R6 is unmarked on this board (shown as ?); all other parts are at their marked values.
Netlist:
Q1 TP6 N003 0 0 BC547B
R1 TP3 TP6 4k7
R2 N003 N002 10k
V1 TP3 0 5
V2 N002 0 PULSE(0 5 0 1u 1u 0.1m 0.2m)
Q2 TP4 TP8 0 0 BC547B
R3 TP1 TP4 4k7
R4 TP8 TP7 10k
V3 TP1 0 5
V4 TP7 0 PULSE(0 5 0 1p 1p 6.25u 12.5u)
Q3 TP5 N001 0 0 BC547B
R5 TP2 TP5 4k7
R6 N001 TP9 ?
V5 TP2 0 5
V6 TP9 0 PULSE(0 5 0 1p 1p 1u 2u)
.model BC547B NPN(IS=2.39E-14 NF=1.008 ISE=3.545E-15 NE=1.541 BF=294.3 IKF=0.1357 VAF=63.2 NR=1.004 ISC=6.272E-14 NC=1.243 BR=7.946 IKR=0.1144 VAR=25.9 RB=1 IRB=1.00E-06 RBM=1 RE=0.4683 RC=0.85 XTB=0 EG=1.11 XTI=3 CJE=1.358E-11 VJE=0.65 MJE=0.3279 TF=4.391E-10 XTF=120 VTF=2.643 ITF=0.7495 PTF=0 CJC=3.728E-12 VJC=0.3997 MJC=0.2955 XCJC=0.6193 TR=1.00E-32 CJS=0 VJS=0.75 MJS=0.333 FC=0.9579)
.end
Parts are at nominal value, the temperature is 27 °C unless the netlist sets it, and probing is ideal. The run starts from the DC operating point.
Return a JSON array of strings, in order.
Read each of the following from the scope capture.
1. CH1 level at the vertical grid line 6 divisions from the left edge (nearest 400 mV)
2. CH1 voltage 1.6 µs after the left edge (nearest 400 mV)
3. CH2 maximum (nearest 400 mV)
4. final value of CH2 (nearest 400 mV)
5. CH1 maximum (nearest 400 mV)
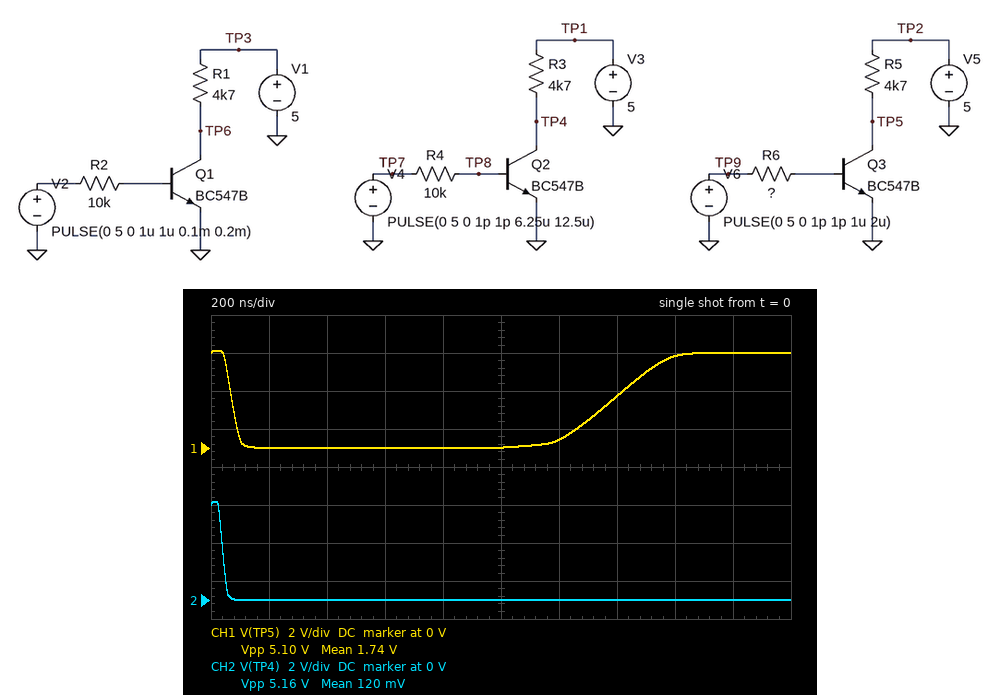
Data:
["400 mV", "4.8 V", "5.2 V", "0 V", "5.2 V"]
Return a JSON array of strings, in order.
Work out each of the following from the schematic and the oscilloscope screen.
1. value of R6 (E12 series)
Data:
["18 kΩ"]
